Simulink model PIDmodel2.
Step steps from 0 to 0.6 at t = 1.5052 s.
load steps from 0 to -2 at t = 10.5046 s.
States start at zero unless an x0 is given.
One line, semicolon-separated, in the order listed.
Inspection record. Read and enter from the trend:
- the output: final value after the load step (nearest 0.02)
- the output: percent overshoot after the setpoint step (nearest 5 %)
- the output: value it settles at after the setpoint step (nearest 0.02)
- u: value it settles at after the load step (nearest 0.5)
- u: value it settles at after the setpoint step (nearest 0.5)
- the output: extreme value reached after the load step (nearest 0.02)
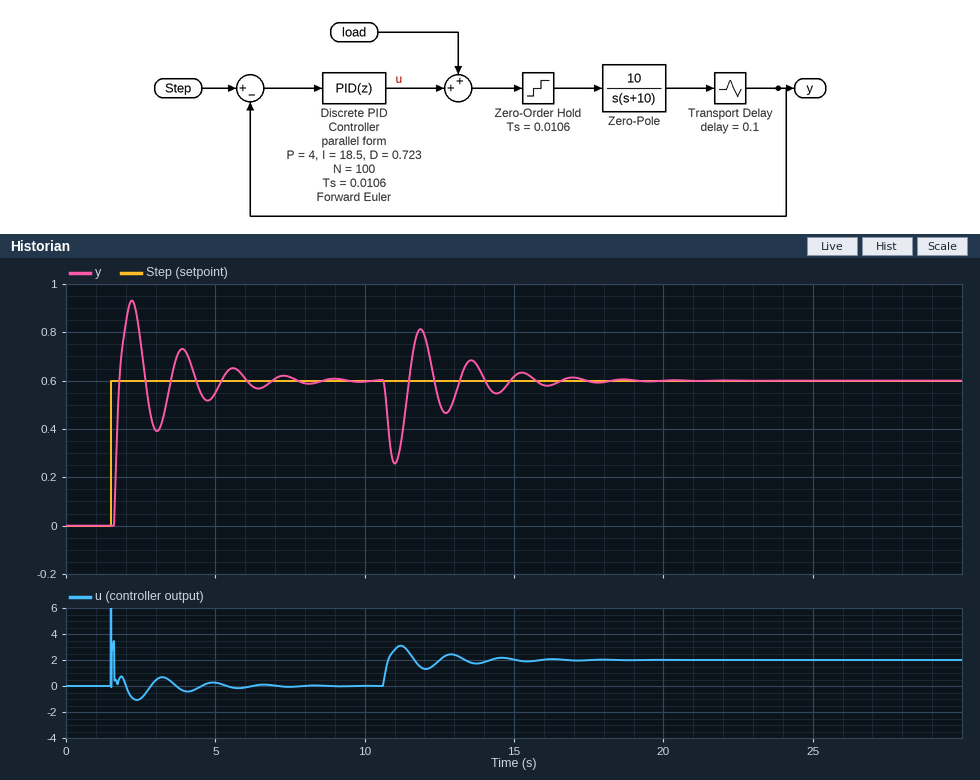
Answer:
0.60; 55 %; 0.60; 2.0; 0.0; 0.26
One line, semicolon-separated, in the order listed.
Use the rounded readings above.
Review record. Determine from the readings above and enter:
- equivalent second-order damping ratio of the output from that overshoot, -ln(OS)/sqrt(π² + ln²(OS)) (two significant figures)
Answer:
0.19
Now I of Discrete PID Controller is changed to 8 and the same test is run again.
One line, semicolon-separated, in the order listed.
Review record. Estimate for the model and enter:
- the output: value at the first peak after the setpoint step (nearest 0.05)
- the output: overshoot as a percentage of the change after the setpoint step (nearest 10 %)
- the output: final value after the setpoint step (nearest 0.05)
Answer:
0.75; 30 %; 0.60
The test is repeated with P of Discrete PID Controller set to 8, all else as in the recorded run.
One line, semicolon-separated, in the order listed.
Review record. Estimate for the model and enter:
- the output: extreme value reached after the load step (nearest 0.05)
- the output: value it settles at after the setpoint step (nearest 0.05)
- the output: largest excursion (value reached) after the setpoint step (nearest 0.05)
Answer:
0.30; 0.60; 1.00
